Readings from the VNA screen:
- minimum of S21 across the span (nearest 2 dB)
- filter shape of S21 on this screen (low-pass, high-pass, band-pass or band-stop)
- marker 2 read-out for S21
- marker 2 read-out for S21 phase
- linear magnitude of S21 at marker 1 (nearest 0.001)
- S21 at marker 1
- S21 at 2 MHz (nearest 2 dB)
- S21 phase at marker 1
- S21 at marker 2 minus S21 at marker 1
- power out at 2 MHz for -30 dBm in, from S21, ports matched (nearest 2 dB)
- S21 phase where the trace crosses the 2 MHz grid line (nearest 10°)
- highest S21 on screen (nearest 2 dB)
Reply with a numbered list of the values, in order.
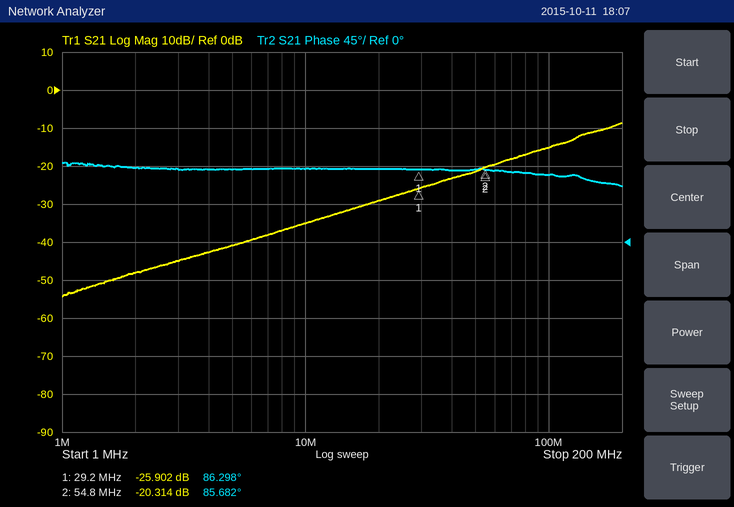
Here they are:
1. -54 dB
2. high-pass
3. -20.314 dB
4. 85.682°
5. 0.051
6. -25.902 dB
7. -48 dB
8. 86.298°
9. 5.588 dB
10. -78 dBm
11. 90°
12. -8 dB
